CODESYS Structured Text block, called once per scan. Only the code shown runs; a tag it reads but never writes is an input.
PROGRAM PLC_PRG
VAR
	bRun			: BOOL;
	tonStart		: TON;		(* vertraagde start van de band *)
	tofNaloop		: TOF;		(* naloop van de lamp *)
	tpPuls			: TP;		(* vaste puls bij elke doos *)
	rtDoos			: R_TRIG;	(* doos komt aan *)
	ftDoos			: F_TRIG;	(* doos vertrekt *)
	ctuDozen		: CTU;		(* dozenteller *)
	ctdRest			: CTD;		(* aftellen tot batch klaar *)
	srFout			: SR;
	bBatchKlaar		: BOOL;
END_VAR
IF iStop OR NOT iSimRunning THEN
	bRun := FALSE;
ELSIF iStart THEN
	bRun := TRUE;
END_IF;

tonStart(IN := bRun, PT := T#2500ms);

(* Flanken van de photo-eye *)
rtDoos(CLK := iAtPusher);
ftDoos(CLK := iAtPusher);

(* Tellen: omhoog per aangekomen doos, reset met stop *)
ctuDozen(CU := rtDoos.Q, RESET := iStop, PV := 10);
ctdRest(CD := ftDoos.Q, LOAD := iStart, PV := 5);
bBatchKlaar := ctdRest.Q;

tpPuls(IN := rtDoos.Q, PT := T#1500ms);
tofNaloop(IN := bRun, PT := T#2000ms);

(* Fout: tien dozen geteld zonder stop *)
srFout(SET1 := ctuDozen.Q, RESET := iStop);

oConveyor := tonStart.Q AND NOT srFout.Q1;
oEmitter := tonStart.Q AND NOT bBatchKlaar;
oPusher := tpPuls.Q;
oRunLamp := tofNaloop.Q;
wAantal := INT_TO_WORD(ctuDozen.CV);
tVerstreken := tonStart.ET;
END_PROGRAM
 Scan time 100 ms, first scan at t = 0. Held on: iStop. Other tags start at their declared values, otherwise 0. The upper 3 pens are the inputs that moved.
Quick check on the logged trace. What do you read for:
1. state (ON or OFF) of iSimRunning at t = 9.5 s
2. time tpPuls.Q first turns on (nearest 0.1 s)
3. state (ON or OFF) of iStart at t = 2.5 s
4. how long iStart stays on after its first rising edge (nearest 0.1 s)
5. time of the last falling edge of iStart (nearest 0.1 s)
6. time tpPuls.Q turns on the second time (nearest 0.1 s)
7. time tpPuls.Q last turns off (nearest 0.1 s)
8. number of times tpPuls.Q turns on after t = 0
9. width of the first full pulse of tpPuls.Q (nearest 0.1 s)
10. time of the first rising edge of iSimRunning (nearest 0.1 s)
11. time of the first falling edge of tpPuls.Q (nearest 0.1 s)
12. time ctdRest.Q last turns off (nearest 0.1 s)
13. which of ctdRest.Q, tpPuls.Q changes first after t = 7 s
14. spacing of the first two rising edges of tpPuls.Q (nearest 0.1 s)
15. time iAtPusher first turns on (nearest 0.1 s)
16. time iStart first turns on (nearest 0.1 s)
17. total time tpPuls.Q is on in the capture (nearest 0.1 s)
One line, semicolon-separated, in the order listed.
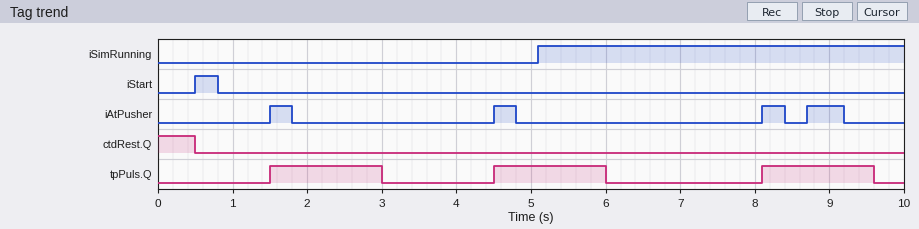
ON; 1.5 s; OFF; 0.3 s; 0.8 s; 4.5 s; 9.6 s; 3; 1.5 s; 5.1 s; 3.0 s; 0.5 s; tpPuls.Q; 3.0 s; 1.5 s; 0.5 s; 4.5 s
